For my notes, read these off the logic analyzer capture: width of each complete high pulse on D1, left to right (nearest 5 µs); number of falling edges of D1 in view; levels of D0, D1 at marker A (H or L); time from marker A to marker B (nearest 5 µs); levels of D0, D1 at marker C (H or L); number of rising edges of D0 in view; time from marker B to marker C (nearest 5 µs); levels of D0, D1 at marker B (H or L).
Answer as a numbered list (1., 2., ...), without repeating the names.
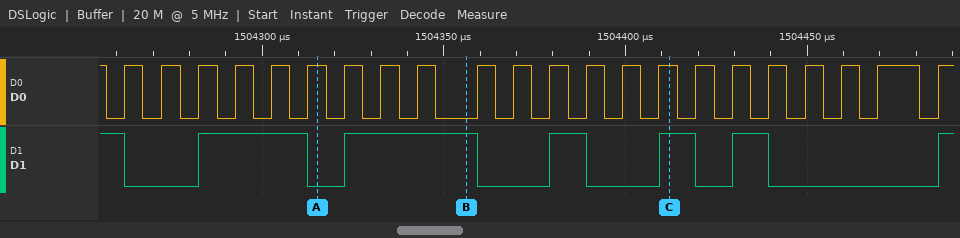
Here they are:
1. 30 µs, 35 µs, 10 µs, 10 µs, 10 µs
2. 6
3. D0=H, D1=L
4. 40 µs
5. D0=H, D1=H
6. 22
7. 55 µs
8. D0=L, D1=H
